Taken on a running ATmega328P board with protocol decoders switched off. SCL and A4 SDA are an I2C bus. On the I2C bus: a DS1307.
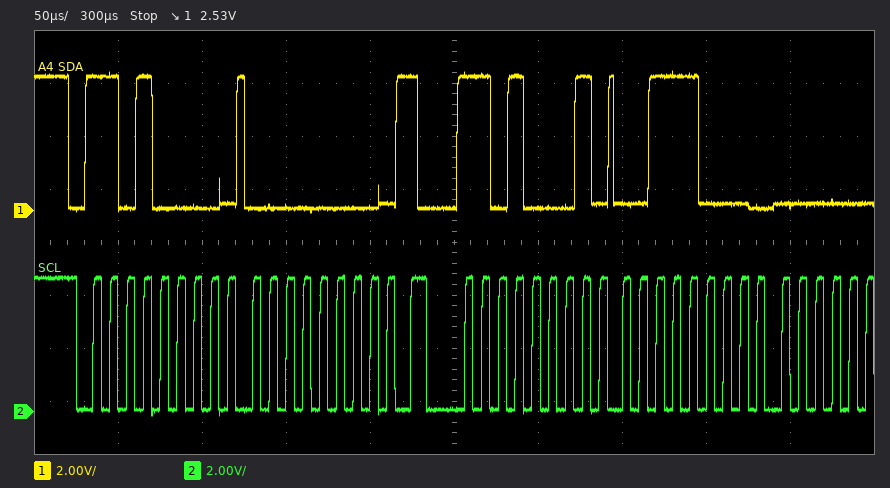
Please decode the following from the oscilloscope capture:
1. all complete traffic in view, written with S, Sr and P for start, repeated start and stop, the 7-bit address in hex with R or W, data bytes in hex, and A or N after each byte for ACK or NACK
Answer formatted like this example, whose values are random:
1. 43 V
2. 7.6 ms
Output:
1. S 68W A 00 A Sr 68R A 38 A
